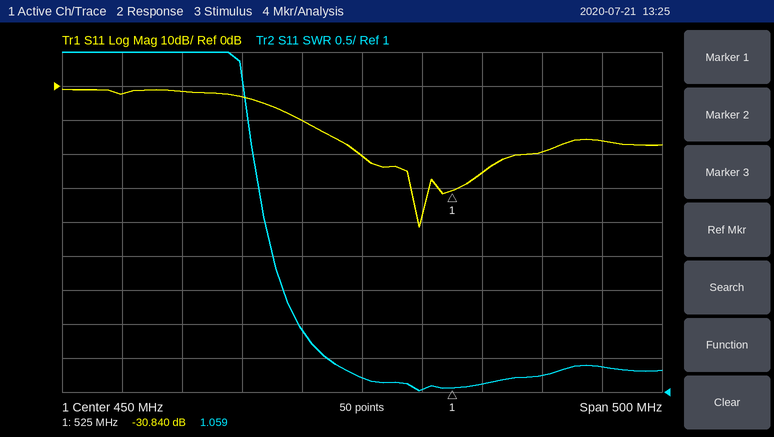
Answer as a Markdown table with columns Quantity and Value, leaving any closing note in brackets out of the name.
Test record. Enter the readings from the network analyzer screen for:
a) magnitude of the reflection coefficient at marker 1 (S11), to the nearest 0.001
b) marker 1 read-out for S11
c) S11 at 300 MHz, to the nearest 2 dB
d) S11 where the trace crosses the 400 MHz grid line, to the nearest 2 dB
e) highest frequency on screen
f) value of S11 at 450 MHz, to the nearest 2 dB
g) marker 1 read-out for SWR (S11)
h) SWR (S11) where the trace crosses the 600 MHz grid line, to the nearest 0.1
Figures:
| Quantity | Value |
|---|---|
| magnitude of the reflection coefficient at marker 1 (S11), to the nearest 0.001 | 0.029 |
| marker 1 read-out for S11 | -30.840 dB |
| S11 at 300 MHz, to the nearest 2 dB | -2 dB |
| S11 where the trace crosses the 400 MHz grid line, to the nearest 2 dB | -10 dB |
| highest frequency on screen | 700 MHz |
| value of S11 at 450 MHz, to the nearest 2 dB | -20 dB |
| marker 1 read-out for SWR | 1.059 |
| SWR (S11) where the trace crosses the 600 MHz grid line, to the nearest 0.1 | 1.2 |
